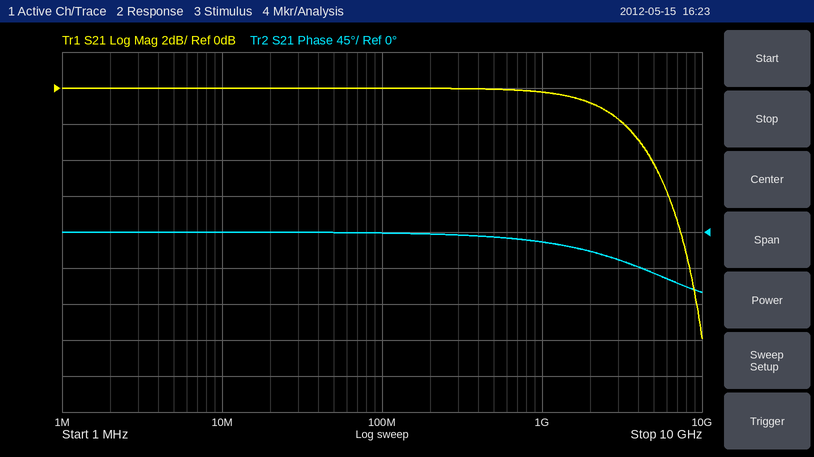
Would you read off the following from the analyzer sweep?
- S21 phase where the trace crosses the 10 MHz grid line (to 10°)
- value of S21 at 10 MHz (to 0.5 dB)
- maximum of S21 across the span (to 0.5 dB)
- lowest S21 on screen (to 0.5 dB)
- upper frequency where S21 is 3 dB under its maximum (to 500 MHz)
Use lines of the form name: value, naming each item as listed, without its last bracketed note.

S21 phase where the trace crosses the 10 MHz grid line: 0°
value of S21 at 10 MHz: 0.0 dB
maximum of S21 across the span: 0.0 dB
lowest S21 on screen: -14.0 dB
upper frequency where S21 is 3 dB under its maximum: 4.0 GHz
